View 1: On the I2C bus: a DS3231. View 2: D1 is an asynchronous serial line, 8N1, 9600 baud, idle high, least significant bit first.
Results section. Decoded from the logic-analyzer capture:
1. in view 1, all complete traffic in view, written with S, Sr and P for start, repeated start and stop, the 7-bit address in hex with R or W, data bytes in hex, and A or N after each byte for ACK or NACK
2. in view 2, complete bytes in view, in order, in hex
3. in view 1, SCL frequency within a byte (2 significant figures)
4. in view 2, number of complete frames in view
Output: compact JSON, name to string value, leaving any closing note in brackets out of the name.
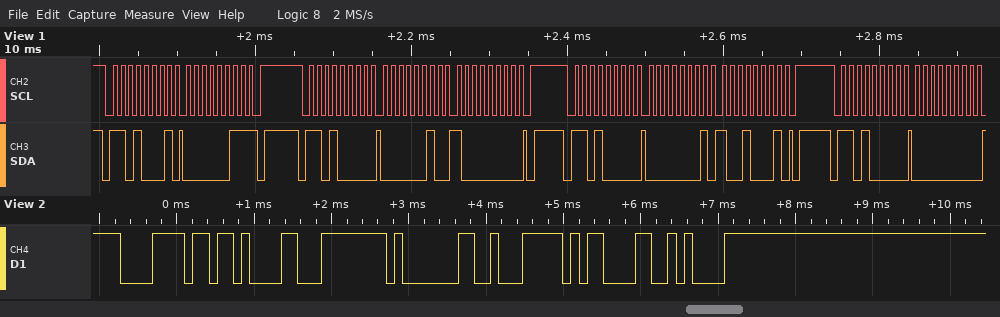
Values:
{"in view 1, all complete traffic in view, written with S, Sr and P for start, repeated start and stop, the 7-bit address in hex with R or W, data bytes in hex, and A or N after each byte for ACK or NACK": "S 68R A 03 N P S 68W A 02 A 80 A P S 68W A 01 A 91 A P S 68W A 00 A", "in view 2, complete bytes in view, in order, in hex": "0x78 0x0B 0xFC 0x01 0xE2 0x0D 0x0A", "in view 1, SCL frequency within a byte": "100 kHz", "in view 2, number of complete frames in view": "7"}
